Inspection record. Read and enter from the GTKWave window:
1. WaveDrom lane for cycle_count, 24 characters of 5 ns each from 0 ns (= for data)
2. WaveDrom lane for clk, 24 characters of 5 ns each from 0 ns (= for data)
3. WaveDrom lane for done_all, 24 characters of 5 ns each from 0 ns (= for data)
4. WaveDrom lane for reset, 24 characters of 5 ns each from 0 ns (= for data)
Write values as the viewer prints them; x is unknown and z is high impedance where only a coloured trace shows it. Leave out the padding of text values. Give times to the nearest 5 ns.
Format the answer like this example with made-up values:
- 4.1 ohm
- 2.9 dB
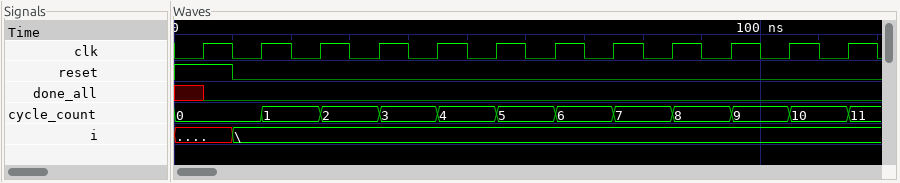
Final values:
- {name: 'cycle_count', wave: '=..=.=.=.=.=.=.=.=.=.=.=', data: '0 1 2 3 4 5 6 7 8 9 10 11'}
- {name: 'clk', wave: '010101010101010101010101'}
- {name: 'done_all', wave: 'x0......................'}
- {name: 'reset', wave: '1.0.....................'}
